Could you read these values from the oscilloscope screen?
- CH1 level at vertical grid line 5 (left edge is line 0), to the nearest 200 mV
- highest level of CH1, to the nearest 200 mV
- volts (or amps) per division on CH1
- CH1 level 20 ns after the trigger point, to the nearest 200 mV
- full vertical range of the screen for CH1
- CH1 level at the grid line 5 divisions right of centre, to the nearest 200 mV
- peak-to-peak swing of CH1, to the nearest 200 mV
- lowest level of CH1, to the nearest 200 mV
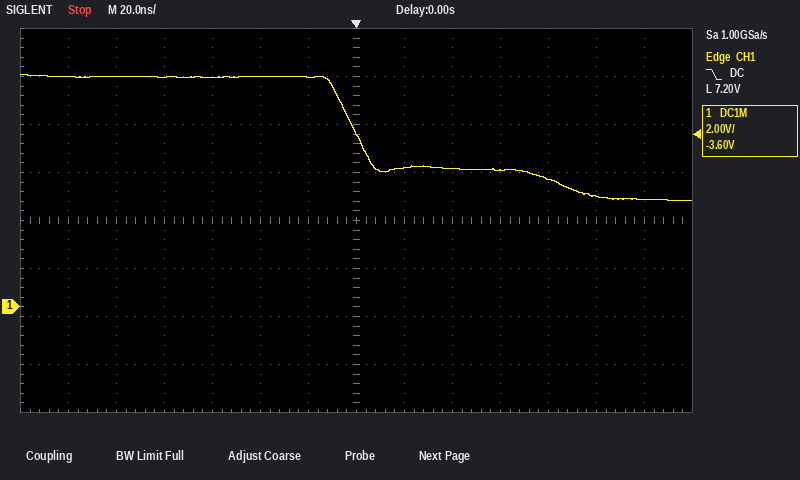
9.6 V
9.6 V
2 V
5.8 V
16 V
4.6 V
5.2 V
4.4 V
